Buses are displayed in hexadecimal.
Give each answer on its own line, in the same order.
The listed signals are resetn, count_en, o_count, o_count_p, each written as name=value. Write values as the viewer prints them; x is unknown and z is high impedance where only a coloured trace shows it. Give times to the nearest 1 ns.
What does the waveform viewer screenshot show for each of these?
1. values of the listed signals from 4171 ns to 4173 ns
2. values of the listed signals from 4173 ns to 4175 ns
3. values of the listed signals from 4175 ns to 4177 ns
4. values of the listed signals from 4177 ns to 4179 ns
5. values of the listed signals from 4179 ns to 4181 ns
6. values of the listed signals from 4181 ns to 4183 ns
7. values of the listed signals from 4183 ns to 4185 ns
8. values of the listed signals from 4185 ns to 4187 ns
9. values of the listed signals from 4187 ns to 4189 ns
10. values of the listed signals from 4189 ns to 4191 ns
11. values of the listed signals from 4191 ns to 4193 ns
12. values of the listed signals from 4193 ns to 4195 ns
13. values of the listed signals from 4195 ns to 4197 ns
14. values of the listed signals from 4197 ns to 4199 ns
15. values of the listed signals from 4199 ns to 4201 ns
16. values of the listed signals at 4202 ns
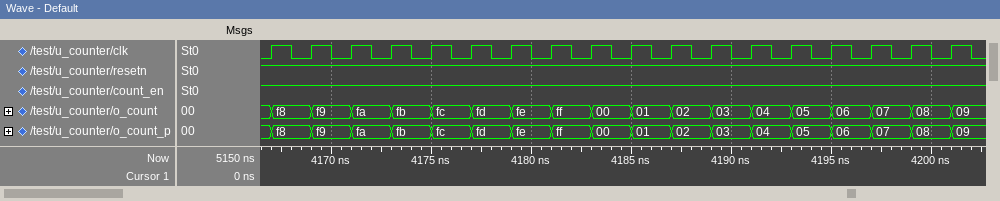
resetn=1, count_en=1, o_count=fa, o_count_p=fa
resetn=1, count_en=1, o_count=fb, o_count_p=fb
resetn=1, count_en=1, o_count=fc, o_count_p=fc
resetn=1, count_en=1, o_count=fd, o_count_p=fd
resetn=1, count_en=1, o_count=fe, o_count_p=fe
resetn=1, count_en=1, o_count=ff, o_count_p=ff
resetn=1, count_en=1, o_count=00, o_count_p=00
resetn=1, count_en=1, o_count=01, o_count_p=01
resetn=1, count_en=1, o_count=02, o_count_p=02
resetn=1, count_en=1, o_count=03, o_count_p=03
resetn=1, count_en=1, o_count=04, o_count_p=04
resetn=1, count_en=1, o_count=05, o_count_p=05
resetn=1, count_en=1, o_count=06, o_count_p=06
resetn=1, count_en=1, o_count=07, o_count_p=07
resetn=1, count_en=1, o_count=08, o_count_p=08
resetn=1, count_en=1, o_count=09, o_count_p=09
